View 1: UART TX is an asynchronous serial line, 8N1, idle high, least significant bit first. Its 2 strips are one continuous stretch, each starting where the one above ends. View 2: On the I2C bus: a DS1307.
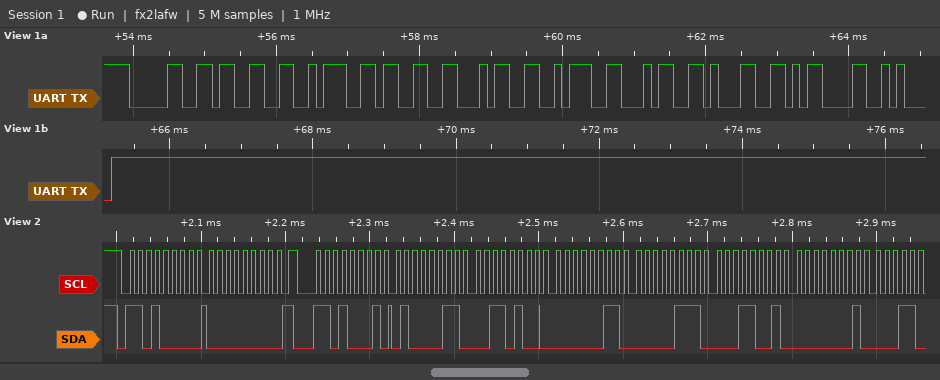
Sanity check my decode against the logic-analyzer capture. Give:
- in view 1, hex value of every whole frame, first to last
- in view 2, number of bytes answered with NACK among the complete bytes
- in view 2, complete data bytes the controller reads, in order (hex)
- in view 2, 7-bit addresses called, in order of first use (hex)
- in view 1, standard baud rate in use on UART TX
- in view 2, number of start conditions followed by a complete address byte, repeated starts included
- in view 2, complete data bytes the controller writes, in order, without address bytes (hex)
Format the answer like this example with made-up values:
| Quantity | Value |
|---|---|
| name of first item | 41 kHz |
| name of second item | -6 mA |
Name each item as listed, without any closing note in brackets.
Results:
| Quantity | Value |
|---|---|
| in view 1, hex value of every whole frame, first to last | 30 33 3A 33 34 3A 34 31 0D 0A |
| in view 2, number of bytes answered with NACK among the complete bytes | 0 |
| in view 2, complete data bytes the controller reads, in order | 43 34 03 07 19 01 |
| in view 2, 7-bit addresses called, in order of first use | 0x68 |
| in view 1, standard baud rate in use on UART TX | 9600 baud |
| in view 2, number of start conditions followed by a complete address byte, repeated starts included | 2 |
| in view 2, complete data bytes the controller writes, in order, without address bytes | 00 |
